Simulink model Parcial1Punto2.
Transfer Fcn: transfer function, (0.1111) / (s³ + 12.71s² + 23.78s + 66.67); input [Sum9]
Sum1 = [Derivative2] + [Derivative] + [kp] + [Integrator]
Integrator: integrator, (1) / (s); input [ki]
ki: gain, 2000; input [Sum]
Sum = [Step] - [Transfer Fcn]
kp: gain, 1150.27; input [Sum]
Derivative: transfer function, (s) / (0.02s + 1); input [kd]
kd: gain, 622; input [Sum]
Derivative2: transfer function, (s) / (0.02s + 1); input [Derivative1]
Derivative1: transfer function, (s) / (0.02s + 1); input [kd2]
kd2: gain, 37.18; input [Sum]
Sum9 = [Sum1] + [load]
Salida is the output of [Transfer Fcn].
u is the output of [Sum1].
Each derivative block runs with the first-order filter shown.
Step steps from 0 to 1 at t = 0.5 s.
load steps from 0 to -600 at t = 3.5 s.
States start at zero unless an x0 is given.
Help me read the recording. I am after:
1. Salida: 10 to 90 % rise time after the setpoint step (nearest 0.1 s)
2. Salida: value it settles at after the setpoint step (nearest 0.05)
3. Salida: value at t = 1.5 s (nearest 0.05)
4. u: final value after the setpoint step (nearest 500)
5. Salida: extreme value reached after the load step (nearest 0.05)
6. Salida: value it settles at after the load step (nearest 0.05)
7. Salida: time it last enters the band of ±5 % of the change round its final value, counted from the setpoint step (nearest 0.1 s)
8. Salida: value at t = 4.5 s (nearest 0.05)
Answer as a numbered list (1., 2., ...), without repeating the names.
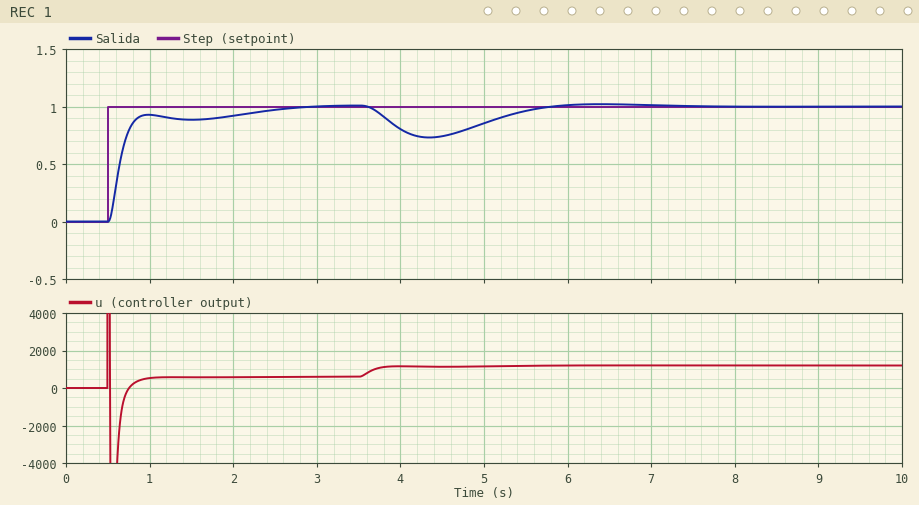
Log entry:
1. 0.3 s
2. 1.00
3. 0.90
4. 500
5. 0.75
6. 1.00
7. 1.8 s
8. 0.75
